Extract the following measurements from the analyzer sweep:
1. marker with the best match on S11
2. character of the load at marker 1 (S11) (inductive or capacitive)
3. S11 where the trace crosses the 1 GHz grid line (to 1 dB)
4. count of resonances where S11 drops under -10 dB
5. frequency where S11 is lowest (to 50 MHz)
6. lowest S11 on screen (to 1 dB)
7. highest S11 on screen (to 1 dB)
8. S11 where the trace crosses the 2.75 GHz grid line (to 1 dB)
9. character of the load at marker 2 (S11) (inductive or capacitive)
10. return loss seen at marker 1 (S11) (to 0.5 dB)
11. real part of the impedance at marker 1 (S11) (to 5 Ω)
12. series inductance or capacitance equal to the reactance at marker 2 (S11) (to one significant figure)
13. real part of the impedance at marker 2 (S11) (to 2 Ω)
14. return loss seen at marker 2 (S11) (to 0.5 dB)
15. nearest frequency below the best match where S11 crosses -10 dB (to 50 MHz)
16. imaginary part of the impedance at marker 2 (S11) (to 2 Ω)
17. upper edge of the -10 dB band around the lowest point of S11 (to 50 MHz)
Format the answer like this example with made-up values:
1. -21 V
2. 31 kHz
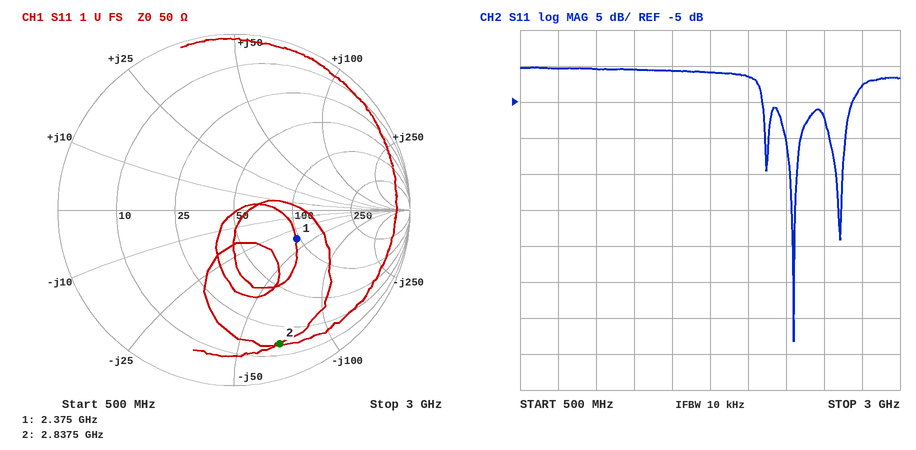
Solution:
1. marker 1
2. capacitive
3. 0 dB
4. 3
5. 2.30 GHz
6. -38 dB
7. 0 dB
8. -3 dB
9. capacitive
10. 8.0 dB
11. 95 Ω
12. 800 fF
13. 16 Ω
14. 2.0 dB
15. 2.25 GHz
16. -68 Ω
17. 2.35 GHz
